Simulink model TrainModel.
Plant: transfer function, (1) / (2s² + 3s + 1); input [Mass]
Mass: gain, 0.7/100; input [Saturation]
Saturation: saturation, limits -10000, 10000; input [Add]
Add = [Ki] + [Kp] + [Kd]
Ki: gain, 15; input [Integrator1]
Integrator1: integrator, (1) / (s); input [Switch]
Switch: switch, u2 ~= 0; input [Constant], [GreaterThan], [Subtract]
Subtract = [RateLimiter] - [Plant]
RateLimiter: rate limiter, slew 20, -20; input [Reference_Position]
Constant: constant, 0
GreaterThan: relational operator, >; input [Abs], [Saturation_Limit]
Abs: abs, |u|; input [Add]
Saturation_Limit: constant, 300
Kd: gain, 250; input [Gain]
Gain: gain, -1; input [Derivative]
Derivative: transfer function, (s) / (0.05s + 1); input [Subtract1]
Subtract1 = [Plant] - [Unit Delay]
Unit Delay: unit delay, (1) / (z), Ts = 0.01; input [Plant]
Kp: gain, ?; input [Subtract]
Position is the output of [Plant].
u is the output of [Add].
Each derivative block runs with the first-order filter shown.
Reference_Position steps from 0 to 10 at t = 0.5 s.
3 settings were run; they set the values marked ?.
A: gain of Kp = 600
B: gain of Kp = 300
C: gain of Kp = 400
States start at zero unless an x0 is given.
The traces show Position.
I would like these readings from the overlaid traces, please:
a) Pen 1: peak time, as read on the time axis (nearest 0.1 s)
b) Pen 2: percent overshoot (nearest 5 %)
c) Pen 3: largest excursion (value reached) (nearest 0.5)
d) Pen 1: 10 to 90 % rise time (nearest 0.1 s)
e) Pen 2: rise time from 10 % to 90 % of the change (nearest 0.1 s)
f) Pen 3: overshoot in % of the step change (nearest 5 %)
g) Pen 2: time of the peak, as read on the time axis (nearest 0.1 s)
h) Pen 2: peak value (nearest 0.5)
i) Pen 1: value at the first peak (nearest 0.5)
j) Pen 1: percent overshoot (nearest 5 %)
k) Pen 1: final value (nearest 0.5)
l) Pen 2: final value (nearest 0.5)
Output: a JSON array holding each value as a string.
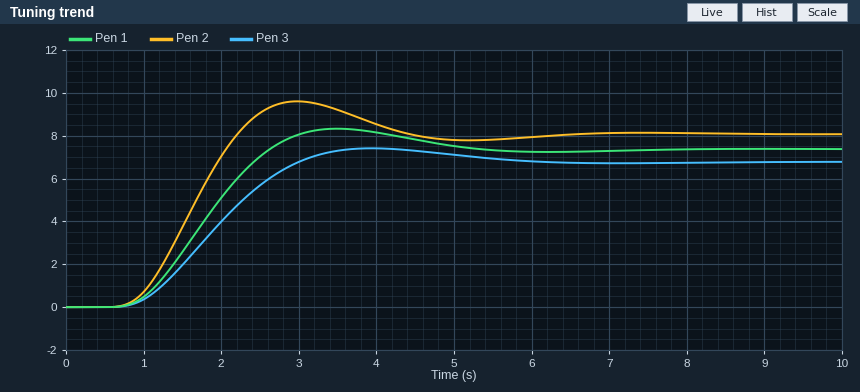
["3.5 s", "20 %", "7.5", "1.3 s", "1.0 s", "10 %", "3.0 s", "9.5", "8.5", "15 %", "7.5", "8.0"]
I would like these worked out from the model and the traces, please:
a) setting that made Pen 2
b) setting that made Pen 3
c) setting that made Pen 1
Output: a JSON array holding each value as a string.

["A", "B", "C"]
